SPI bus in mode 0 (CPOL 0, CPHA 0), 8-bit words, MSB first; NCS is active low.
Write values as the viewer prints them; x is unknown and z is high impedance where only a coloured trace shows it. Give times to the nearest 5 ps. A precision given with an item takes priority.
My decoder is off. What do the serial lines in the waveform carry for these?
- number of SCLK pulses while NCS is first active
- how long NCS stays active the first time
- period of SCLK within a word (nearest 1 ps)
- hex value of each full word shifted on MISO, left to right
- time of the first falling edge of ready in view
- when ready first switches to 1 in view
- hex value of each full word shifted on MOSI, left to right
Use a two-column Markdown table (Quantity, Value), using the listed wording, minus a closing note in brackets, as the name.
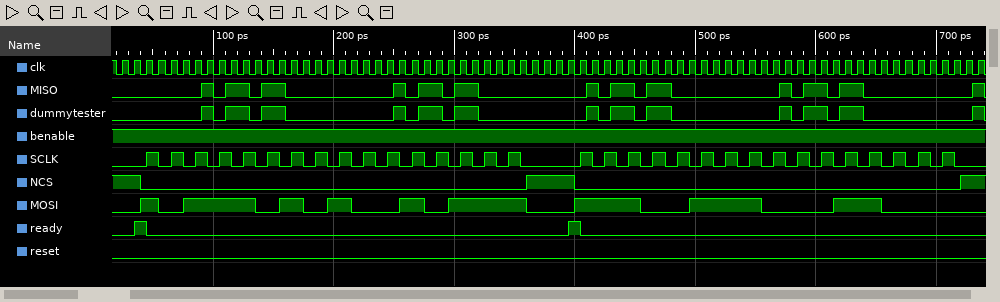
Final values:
| Quantity | Value |
|---|---|
| number of SCLK pulses while NCS is first active | 16 |
| how long NCS stays active the first time | 320 ps |
| period of SCLK within a word | 20 ps |
| hex value of each full word shifted on MISO, left to right | 0C, 0C, 30, 30 |
| time of the first falling edge of ready in view | 45 ps |
| when ready first switches to 1 in view | 35 ps |
| hex value of each full word shifted on MOSI, left to right | BA, 97, E7, 18 |
